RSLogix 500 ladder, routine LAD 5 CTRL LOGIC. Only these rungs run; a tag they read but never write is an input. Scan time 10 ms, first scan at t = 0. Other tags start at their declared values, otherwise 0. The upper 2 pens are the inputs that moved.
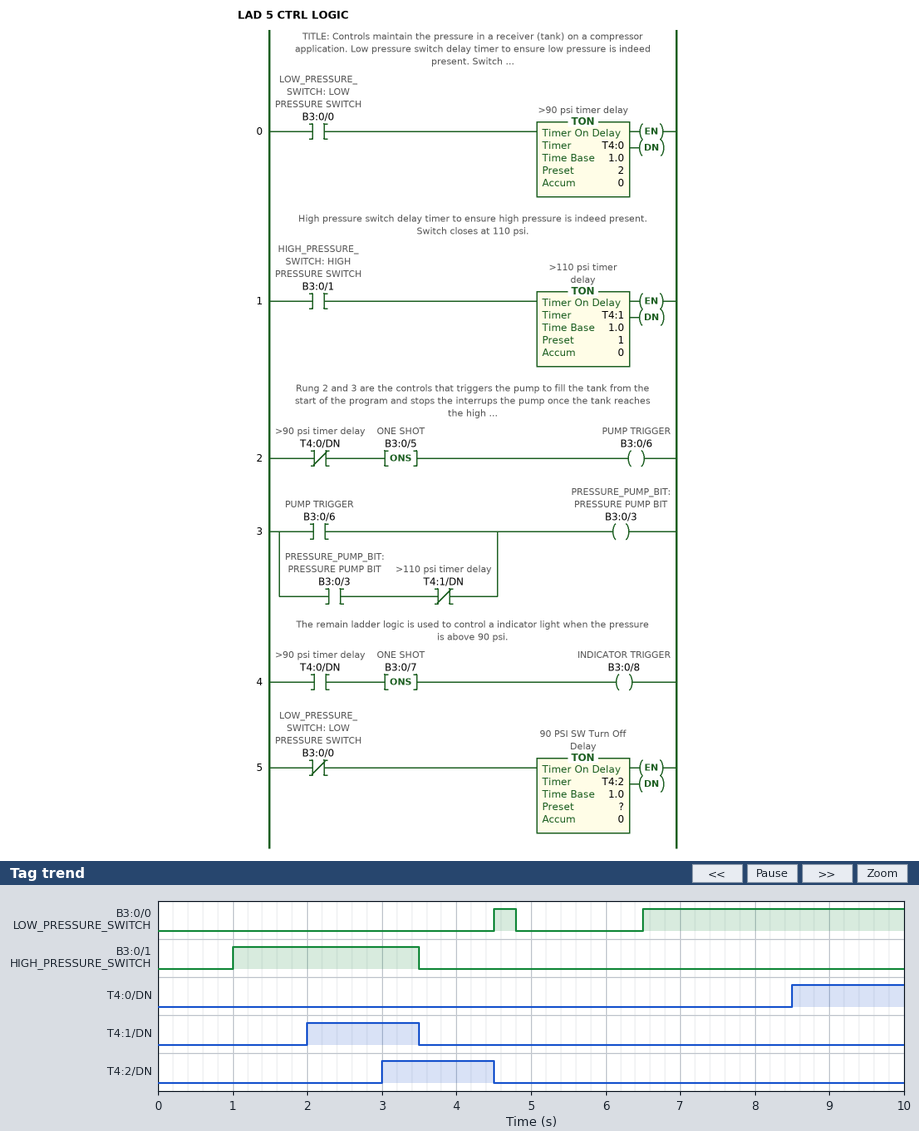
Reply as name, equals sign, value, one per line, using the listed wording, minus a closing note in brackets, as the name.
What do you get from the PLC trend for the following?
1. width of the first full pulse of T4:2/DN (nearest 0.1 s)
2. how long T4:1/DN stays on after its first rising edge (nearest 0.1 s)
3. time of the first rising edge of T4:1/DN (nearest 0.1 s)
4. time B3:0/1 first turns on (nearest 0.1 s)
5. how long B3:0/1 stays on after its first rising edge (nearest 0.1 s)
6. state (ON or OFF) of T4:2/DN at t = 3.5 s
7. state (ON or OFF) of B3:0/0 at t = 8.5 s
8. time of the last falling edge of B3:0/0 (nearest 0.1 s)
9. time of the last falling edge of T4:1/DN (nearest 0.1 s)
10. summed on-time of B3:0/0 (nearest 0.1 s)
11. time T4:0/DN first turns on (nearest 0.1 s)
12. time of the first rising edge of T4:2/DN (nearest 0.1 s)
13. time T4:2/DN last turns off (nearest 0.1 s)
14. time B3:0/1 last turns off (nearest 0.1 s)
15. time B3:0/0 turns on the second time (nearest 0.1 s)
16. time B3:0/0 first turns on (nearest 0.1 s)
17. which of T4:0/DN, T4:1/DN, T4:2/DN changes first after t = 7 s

width of the first full pulse of T4:2/DN = 1.5 s
how long T4:1/DN stays on after its first rising edge = 1.5 s
time of the first rising edge of T4:1/DN = 2.0 s
time B3:0/1 first turns on = 1.0 s
how long B3:0/1 stays on after its first rising edge = 2.5 s
state (ON or OFF) of T4:2/DN at t = 3.5 s = ON
state (ON or OFF) of B3:0/0 at t = 8.5 s = ON
time of the last falling edge of B3:0/0 = 4.8 s
time of the last falling edge of T4:1/DN = 3.5 s
summed on-time of B3:0/0 = 3.8 s
time T4:0/DN first turns on = 8.5 s
time of the first rising edge of T4:2/DN = 3.0 s
time T4:2/DN last turns off = 4.5 s
time B3:0/1 last turns off = 3.5 s
time B3:0/0 turns on the second time = 6.5 s
time B3:0/0 first turns on = 4.5 s
which of T4:0/DN, T4:1/DN, T4:2/DN changes first after t = 7 s = T4:0/DN
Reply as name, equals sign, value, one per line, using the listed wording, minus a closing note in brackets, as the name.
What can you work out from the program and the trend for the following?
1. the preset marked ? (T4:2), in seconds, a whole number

the preset marked ? (T4:2), in seconds, a whole number = 3 s
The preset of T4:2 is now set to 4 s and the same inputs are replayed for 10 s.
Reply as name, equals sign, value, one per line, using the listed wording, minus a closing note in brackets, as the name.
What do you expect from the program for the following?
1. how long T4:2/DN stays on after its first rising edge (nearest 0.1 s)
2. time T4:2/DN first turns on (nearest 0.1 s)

how long T4:2/DN stays on after its first rising edge = 0.5 s
time T4:2/DN first turns on = 4.0 s
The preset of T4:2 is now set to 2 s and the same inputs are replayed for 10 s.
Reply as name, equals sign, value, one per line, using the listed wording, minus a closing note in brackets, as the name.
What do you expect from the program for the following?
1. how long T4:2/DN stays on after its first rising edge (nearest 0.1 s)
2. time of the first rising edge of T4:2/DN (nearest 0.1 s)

how long T4:2/DN stays on after its first rising edge = 2.5 s
time of the first rising edge of T4:2/DN = 2.0 s
